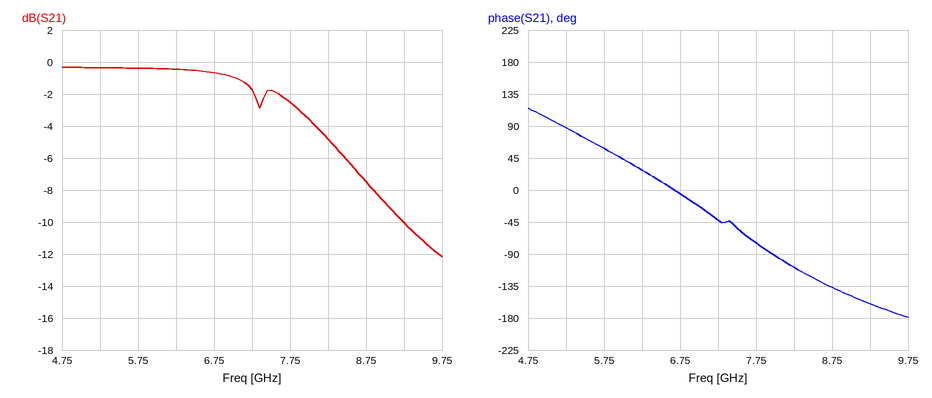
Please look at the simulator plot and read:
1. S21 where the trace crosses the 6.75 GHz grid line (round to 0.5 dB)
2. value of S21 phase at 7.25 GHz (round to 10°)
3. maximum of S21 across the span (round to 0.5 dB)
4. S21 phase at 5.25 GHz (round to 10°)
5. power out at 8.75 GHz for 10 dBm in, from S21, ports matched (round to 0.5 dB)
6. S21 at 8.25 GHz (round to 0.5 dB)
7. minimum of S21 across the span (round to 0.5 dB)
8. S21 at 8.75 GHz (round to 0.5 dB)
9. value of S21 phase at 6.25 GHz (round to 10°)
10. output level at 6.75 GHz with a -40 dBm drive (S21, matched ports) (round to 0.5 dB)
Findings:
-0.5 dB
-40°
-0.5 dB
90°
2.5 dBm
-5.0 dB
-12.0 dB
-7.5 dB
30°
-40.5 dBm
